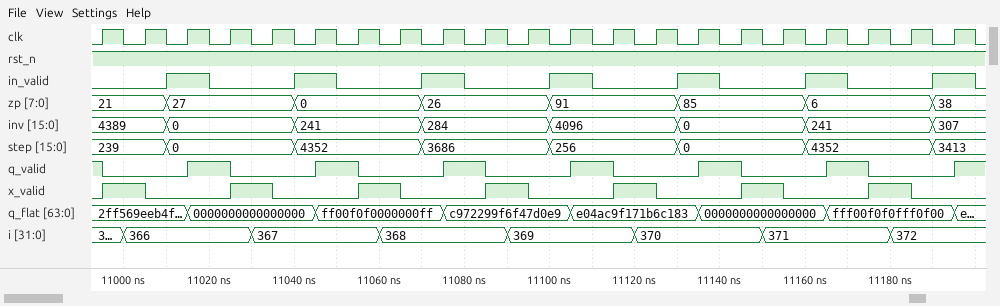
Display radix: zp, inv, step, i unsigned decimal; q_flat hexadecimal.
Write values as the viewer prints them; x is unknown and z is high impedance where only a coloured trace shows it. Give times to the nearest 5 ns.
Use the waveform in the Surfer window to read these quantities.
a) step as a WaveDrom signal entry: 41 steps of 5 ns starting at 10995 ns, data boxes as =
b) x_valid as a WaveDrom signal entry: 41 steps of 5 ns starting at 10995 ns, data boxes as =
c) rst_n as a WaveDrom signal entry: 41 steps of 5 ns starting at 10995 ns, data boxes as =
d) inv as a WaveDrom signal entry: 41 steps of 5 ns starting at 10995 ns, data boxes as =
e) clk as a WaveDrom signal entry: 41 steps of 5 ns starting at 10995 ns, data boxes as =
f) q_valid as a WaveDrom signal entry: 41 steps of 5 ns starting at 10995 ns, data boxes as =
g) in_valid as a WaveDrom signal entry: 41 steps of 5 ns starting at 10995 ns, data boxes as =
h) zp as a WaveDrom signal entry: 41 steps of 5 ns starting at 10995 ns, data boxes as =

{name: 'step', wave: '=..=.....=.....=.....=.....=.....=.....=.', data: '239 0 4352 3686 256 0 4352 3413'}
{name: 'x_valid', wave: '1.0...1.0...1.0...1.0...1.0...1.0...1.0..'}
{name: 'rst_n', wave: '1........................................'}
{name: 'inv', wave: '=..=.....=.....=.....=.....=.....=.....=.', data: '4389 0 241 284 4096 0 241 307'}
{name: 'clk', wave: '10101010101010101010101010101010101010101'}
{name: 'q_valid', wave: '0...1.0...1.0...1.0...1.0...1.0...1.0...1'}
{name: 'in_valid', wave: '0..1.0...1.0...1.0...1.0...1.0...1.0...1.'}
{name: 'zp', wave: '=..=.....=.....=.....=.....=.....=.....=.', data: '21 27 0 26 91 85 6 38'}
